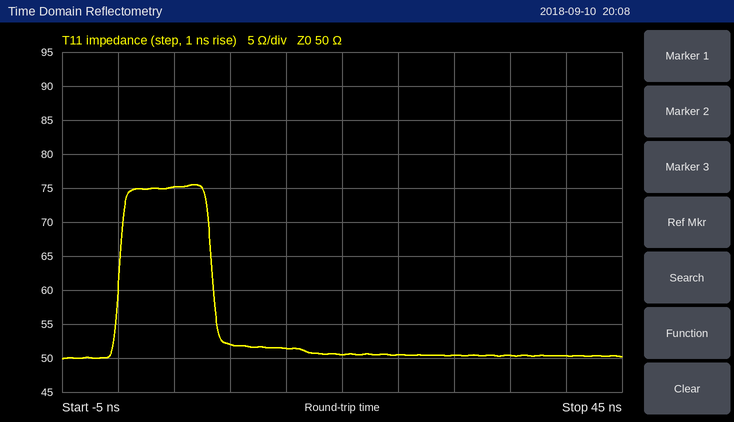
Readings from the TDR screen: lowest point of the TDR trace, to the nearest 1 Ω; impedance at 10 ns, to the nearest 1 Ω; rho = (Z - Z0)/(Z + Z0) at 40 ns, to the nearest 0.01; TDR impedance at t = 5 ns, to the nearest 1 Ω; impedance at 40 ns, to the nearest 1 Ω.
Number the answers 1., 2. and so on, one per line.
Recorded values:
1. 50 Ω
2. 52 Ω
3. 0.00
4. 75 Ω
5. 50 Ω
